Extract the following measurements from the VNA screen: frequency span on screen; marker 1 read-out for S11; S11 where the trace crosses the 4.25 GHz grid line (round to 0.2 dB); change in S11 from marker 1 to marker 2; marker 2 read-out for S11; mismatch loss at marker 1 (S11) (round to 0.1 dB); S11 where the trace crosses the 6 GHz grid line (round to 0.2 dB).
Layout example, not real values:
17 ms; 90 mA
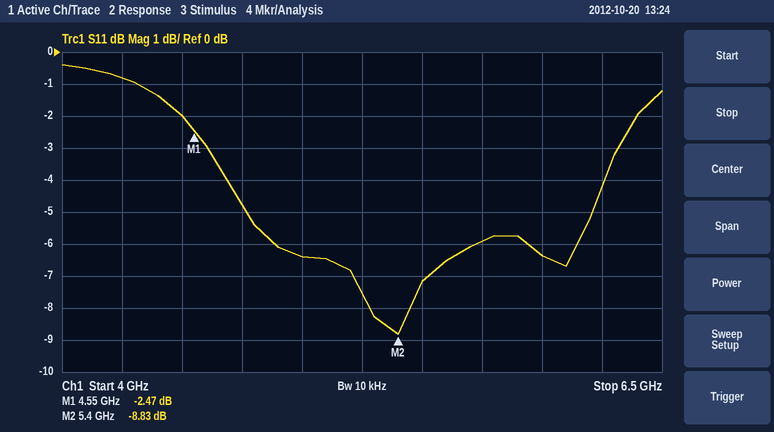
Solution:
2.5 GHz; -2.47 dB; -0.8 dB; -6.36 dB; -8.83 dB; 3.6 dB; -6.4 dB
